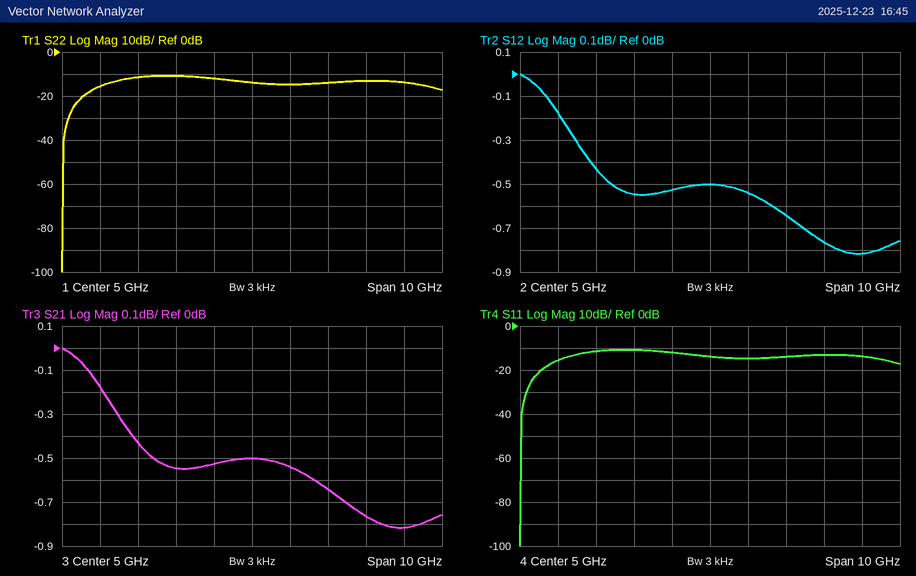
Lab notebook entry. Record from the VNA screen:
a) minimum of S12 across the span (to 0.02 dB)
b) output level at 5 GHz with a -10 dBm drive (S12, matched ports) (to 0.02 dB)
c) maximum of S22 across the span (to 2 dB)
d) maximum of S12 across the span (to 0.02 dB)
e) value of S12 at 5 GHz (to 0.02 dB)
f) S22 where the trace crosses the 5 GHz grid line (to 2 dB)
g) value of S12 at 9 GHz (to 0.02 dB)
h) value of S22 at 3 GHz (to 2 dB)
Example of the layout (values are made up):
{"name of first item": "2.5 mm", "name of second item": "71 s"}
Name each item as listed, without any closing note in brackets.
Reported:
{"minimum of S12 across the span": "-0.82 dB", "output level at 5 GHz with a -10 dBm drive (S12, matched ports)": "-10.50 dBm", "maximum of S22 across the span": "-10 dB", "maximum of S12 across the span": "0.00 dB", "value of S12 at 5 GHz": "-0.50 dB", "S22 where the trace crosses the 5 GHz grid line": "-14 dB", "value of S12 at 9 GHz": "-0.82 dB", "value of S22 at 3 GHz": "-10 dB"}
